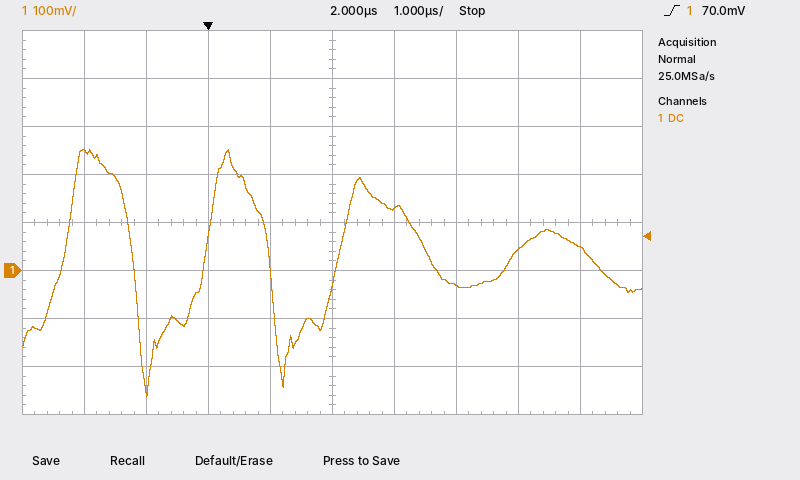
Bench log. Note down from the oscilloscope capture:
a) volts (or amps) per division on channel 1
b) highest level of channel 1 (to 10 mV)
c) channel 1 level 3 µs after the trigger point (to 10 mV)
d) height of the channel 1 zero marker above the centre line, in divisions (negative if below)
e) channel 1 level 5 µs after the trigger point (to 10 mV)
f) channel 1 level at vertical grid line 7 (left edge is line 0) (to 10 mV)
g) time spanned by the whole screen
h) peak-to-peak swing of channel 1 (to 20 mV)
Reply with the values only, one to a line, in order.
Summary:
100 mV
250 mV
130 mV
-1.0 div
40 mV
-30 mV
10 µs
520 mV
